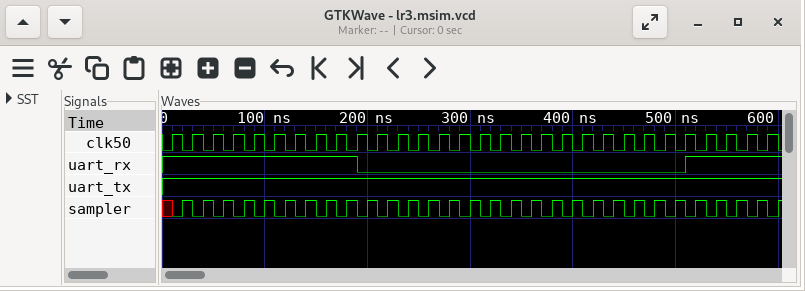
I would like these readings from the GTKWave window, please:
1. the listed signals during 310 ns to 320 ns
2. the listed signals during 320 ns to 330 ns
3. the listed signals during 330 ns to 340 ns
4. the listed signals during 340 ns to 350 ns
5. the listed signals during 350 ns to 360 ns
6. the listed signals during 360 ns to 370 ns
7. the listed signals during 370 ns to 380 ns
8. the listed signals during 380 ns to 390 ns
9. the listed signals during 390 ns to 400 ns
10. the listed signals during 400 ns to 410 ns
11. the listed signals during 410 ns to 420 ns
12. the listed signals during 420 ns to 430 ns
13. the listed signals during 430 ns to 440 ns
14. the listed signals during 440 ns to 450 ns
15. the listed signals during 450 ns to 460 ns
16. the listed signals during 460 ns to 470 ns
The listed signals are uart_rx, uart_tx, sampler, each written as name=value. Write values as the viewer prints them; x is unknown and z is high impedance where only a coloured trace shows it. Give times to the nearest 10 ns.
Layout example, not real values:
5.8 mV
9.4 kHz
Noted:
uart_rx=0, uart_tx=1, sampler=0
uart_rx=0, uart_tx=1, sampler=1
uart_rx=0, uart_tx=1, sampler=0
uart_rx=0, uart_tx=1, sampler=1
uart_rx=0, uart_tx=1, sampler=0
uart_rx=0, uart_tx=1, sampler=1
uart_rx=0, uart_tx=1, sampler=0
uart_rx=0, uart_tx=1, sampler=1
uart_rx=0, uart_tx=1, sampler=0
uart_rx=0, uart_tx=1, sampler=1
uart_rx=0, uart_tx=1, sampler=0
uart_rx=0, uart_tx=1, sampler=1
uart_rx=0, uart_tx=1, sampler=0
uart_rx=0, uart_tx=1, sampler=1
uart_rx=0, uart_tx=1, sampler=0
uart_rx=0, uart_tx=1, sampler=1
